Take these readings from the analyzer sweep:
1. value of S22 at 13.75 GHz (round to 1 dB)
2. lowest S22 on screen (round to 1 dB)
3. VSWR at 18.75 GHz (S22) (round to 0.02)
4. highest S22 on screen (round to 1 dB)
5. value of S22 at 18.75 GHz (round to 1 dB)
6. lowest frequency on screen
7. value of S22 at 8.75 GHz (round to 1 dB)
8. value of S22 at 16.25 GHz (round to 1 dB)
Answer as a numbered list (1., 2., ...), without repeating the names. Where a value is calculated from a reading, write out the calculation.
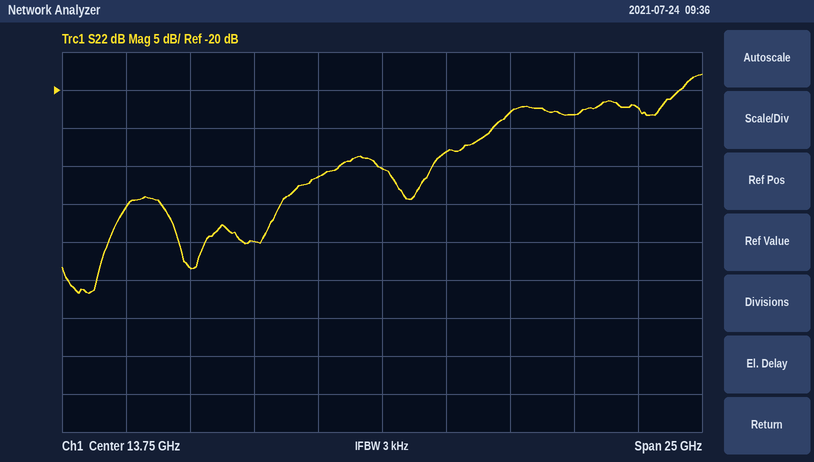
1. -30 dB
2. -47 dB
3. |Γ| = 10^(-23/20) = 0.0708; VSWR = (1 + 0.0708)/(1 − 0.0708) ≈ 1.15, so 1.16 to the nearest 0.02
4. -18 dB
5. -23 dB
6. 1.25 GHz
7. -40 dB
8. -28 dB
